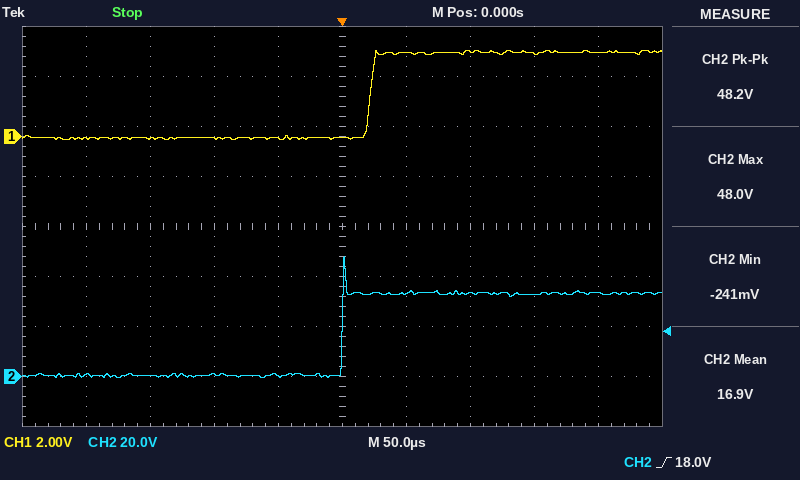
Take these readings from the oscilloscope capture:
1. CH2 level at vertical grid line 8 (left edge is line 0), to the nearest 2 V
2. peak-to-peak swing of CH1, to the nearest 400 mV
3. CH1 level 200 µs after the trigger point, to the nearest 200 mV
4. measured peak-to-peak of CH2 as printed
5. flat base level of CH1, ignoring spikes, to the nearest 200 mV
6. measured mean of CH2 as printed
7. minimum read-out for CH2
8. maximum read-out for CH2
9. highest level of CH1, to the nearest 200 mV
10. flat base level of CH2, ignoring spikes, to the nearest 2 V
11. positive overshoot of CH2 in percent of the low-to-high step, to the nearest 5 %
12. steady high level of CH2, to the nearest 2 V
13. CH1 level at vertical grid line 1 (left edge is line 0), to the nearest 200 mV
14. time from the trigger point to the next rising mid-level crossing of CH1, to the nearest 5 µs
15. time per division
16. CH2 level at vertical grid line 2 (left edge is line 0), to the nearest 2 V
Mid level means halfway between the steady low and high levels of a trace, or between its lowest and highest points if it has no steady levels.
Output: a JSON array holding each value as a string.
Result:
["32 V", "3.6 V", "3.4 V", "48.2 V", "0.0 V", "16.9 V", "-241 mV", "48.0 V", "3.4 V", "0 V", "45 %", "34 V", "0.0 V", "20 µs", "50 µs", "0 V"]
